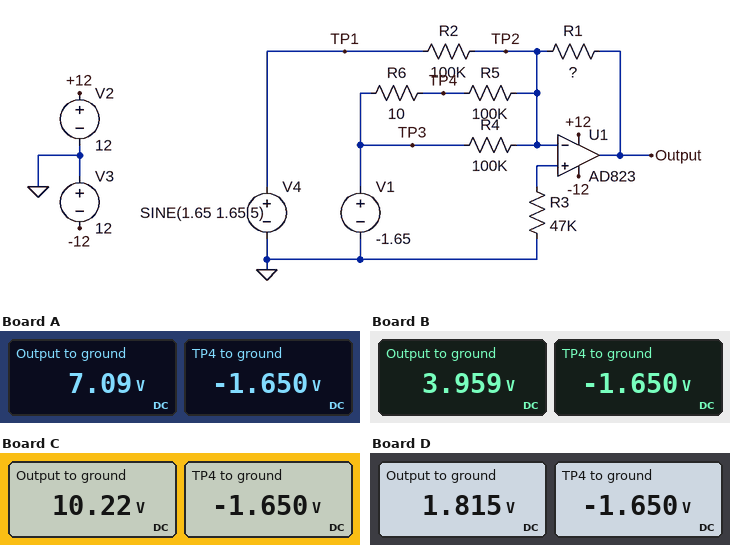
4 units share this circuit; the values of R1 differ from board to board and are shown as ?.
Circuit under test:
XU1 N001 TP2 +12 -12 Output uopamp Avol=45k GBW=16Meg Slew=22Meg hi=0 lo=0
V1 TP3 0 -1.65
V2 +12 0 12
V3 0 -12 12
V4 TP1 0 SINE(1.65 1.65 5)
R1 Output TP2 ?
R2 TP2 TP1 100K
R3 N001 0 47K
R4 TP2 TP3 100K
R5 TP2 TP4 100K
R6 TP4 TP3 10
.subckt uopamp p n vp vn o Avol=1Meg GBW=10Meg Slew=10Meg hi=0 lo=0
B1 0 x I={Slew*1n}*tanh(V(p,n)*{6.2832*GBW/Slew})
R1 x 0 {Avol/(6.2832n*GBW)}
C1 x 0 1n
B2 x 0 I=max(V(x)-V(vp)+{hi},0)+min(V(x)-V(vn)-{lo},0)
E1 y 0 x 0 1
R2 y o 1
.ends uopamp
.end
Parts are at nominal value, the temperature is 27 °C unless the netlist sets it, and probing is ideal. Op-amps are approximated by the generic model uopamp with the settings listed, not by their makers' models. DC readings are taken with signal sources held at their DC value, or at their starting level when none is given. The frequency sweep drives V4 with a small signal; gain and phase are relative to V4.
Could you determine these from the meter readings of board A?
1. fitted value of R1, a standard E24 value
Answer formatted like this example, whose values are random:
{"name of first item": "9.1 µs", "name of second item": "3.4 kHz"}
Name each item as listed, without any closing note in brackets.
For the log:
{"fitted value of R1, a standard E24 value": "430 kΩ"}
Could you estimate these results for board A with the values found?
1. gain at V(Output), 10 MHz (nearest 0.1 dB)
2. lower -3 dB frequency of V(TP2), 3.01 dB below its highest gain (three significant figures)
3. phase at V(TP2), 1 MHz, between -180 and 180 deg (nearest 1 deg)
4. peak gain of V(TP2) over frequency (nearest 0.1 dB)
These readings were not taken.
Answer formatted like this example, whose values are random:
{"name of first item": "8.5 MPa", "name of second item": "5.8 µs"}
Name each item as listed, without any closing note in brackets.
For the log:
{"gain at V(Output), 10 MHz": "-6.2 dB", "lower -3 dB frequency of V(TP2), 3.01 dB below its highest gain": "1.15 MHz", "phase at V(TP2), 1 MHz, between -180 and 180 deg": "49 deg", "peak gain of V(TP2) over frequency": "-10.2 dB"}
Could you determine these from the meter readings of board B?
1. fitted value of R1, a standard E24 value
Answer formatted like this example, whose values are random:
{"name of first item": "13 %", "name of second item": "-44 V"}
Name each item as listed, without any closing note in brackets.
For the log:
{"fitted value of R1, a standard E24 value": "240 kΩ"}
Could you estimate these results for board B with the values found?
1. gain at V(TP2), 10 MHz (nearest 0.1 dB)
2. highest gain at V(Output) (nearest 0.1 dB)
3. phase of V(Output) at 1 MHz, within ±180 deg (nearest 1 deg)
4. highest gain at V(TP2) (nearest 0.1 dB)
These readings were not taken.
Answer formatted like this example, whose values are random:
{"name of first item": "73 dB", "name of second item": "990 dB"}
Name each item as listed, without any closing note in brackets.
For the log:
{"gain at V(TP2), 10 MHz": "-10.8 dB", "highest gain at V(Output)": "7.6 dB", "phase of V(Output) at 1 MHz, within ±180 deg": "153 deg", "highest gain at V(TP2)": "-10.7 dB"}
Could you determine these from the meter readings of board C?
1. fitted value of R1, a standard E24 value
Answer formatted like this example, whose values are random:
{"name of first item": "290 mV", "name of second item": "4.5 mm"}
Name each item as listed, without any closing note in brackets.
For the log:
{"fitted value of R1, a standard E24 value": "620 kΩ"}
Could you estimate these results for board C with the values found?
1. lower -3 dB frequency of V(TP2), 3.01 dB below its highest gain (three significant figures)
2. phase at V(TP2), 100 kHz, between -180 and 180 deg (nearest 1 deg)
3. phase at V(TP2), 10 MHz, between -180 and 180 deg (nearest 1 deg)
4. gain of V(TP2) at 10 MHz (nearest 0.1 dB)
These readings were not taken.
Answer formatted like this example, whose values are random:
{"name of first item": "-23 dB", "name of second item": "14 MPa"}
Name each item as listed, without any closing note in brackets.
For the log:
{"lower -3 dB frequency of V(TP2), 3.01 dB below its highest gain": "817 kHz", "phase at V(TP2), 100 kHz, between -180 and 180 deg": "83 deg", "phase at V(TP2), 10 MHz, between -180 and 180 deg": "5 deg", "gain of V(TP2) at 10 MHz": "-10.0 dB"}
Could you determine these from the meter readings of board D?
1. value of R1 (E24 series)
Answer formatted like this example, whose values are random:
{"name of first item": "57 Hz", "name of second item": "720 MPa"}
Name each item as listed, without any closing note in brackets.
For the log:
{"value of R1": "110 kΩ"}
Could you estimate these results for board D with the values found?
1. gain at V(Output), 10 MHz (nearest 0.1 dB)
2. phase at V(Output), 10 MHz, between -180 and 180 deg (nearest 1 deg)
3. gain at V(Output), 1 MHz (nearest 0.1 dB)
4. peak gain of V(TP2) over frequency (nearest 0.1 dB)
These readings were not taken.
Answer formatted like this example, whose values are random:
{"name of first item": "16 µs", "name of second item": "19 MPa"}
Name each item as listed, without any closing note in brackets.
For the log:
{"gain at V(Output), 10 MHz": "-8.3 dB", "phase at V(Output), 10 MHz, between -180 and 180 deg": "110 deg", "gain at V(Output), 1 MHz": "0.5 dB", "peak gain of V(TP2) over frequency": "-11.8 dB"}
